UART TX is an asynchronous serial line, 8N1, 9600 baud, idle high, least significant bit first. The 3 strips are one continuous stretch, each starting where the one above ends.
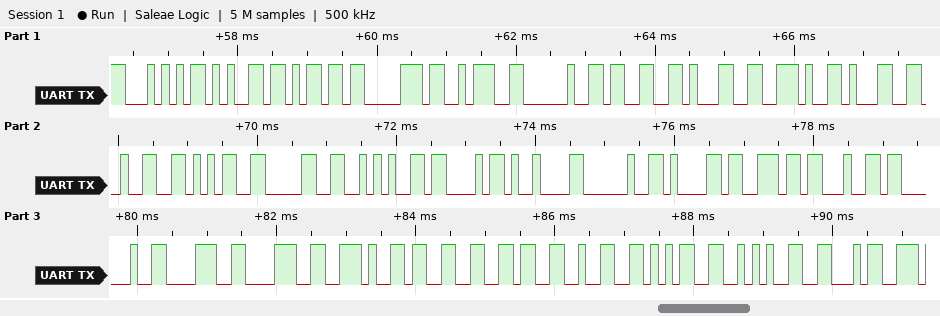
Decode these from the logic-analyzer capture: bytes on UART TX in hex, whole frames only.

54 65 6D 70 3A 20 33 31 2E 31 32 35 30 2A 43 09 20 61 6E 64 20 38 38 2E 33 36 32 35 2A 46
